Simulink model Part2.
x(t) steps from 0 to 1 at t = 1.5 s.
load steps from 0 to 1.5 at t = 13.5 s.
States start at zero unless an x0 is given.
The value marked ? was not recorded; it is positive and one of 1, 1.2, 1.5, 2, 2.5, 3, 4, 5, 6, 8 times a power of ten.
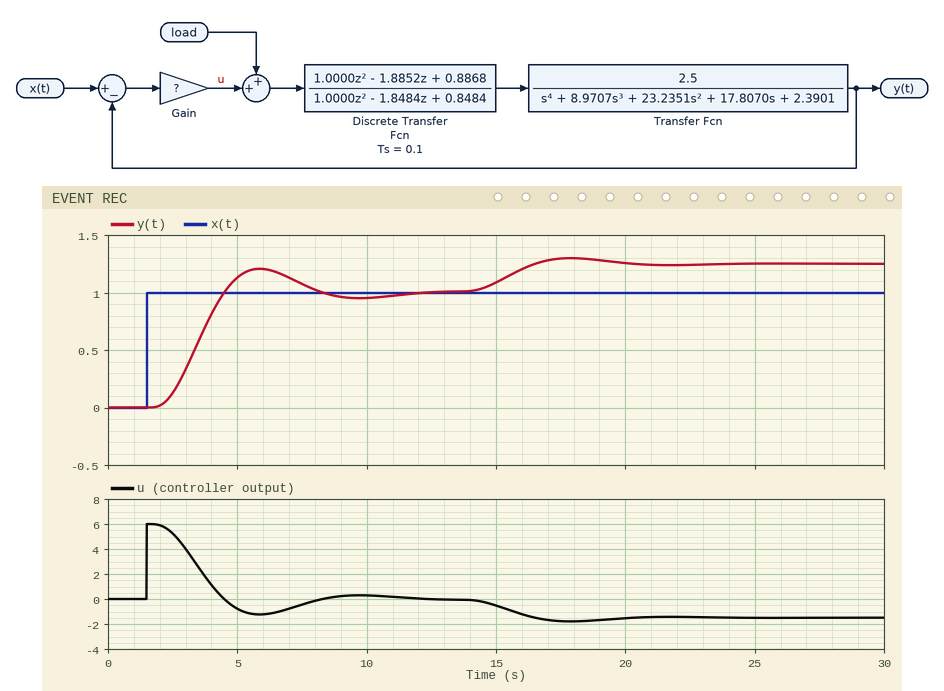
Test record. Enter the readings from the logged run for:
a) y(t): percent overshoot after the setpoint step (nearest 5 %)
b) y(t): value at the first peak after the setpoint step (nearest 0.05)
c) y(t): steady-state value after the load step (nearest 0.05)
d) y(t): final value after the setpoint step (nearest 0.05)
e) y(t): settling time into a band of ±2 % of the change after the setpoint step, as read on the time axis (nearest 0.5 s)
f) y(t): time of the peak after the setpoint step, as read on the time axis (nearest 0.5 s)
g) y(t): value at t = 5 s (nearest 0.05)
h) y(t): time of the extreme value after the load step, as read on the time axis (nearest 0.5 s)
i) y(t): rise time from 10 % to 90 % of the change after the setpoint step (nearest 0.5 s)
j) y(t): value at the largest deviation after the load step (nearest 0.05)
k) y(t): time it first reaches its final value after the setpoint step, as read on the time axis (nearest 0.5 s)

20 %
1.20
1.25
1.00
11.5 s
6.0 s
1.15
18.0 s
2.0 s
1.30
4.5 s
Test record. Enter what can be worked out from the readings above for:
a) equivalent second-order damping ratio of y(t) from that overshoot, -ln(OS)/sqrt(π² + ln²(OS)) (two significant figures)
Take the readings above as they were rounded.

0.46
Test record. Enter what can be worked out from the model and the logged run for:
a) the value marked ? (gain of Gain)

6
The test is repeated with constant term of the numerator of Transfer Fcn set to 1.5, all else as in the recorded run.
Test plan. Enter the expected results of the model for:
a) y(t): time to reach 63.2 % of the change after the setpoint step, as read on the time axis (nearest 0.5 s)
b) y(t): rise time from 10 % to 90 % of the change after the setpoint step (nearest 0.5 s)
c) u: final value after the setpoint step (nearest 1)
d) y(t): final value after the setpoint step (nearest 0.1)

4.5 s
3.0 s
0
1.0
